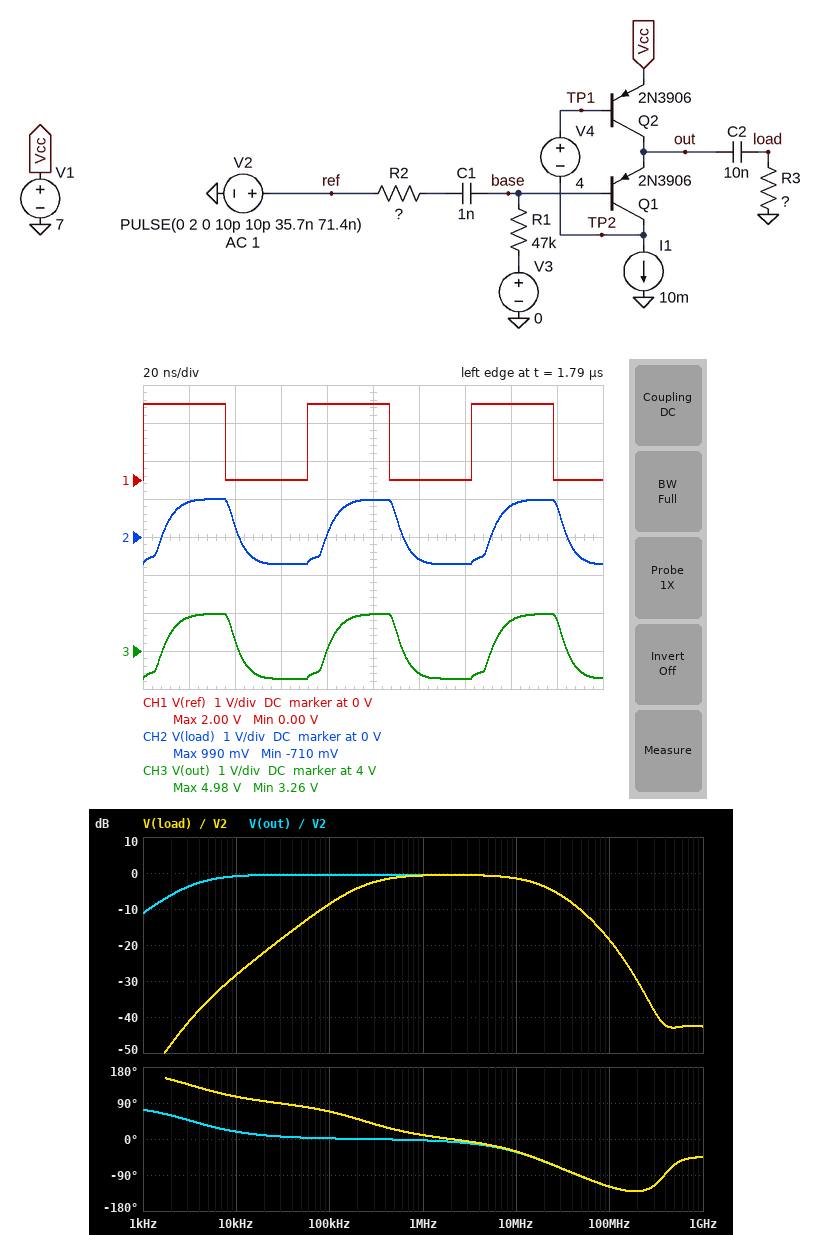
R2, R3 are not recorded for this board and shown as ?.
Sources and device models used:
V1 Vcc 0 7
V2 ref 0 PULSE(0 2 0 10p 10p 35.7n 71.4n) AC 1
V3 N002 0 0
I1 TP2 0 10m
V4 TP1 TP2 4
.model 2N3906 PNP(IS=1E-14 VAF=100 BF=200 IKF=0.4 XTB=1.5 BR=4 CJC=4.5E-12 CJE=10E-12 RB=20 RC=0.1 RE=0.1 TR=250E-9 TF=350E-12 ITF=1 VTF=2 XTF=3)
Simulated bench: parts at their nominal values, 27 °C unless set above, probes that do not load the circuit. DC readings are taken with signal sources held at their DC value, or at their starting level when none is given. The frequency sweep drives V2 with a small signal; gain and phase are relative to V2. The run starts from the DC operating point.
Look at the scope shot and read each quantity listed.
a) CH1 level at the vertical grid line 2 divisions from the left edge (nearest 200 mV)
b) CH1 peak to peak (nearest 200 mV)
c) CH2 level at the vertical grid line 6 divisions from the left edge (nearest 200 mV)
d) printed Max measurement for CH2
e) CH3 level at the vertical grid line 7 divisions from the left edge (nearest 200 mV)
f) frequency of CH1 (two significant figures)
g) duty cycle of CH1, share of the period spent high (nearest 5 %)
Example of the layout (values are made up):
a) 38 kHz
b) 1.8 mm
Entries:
a) 0 V
b) 2.0 V
c) -600 mV
d) 990 mV
e) 3.2 V
f) 14 MHz
g) 50 %
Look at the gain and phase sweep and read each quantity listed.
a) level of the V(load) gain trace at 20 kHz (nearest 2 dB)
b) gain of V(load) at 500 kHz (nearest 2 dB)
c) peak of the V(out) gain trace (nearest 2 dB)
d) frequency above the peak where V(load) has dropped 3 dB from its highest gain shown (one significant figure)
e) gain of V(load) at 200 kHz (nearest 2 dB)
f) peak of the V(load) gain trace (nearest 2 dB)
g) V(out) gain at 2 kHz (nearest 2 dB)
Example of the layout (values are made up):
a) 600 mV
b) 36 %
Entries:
a) -22 dB
b) -2 dB
c) 0 dB
d) 20 MHz
e) -4 dB
f) 0 dB
g) -6 dB
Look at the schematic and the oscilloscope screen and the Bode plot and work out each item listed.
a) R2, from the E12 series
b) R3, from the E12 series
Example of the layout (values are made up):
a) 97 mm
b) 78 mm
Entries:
a) 2.2 kΩ
b) 68 Ω
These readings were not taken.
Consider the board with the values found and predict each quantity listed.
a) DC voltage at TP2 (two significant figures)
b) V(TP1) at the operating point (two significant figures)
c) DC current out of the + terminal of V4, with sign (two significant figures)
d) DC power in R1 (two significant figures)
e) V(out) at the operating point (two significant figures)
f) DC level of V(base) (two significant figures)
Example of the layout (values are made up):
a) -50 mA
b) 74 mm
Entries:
a) 2.3 V
b) 6.3 V
c) -50 µA
d) 120 µW
e) 3.1 V
f) 2.4 V
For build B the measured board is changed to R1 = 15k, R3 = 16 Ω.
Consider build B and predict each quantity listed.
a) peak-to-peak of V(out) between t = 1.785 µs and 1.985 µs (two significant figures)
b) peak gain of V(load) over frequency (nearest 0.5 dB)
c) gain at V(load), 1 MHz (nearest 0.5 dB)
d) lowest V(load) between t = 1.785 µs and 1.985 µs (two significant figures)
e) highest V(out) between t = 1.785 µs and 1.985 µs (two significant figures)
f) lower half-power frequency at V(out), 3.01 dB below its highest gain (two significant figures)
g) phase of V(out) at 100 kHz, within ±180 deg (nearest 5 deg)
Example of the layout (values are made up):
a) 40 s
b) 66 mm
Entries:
a) 860 mV
b) -32.0 dB
c) -34.0 dB
d) -190 mV
e) 3.6 V
f) 39 kHz
g) 5 deg
